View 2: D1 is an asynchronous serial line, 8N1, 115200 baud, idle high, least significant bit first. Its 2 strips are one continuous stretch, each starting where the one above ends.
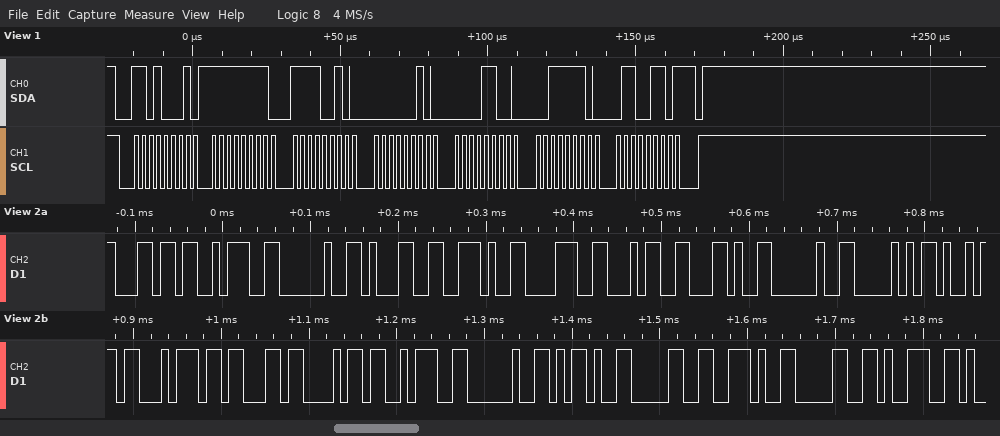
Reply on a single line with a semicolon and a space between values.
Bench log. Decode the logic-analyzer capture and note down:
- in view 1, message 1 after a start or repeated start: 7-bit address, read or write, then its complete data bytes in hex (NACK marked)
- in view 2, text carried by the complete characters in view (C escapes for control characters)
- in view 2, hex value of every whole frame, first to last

0x68 read: FF F2 02 0C 3E 66 NACK; "l: 1.84, Pitch: -0.09"; 0x6C 0x3A 0x20 0x31 0x2E 0x38 0x34 0x2C 0x20 0x50 0x69 0x74 0x63 0x68 0x3A 0x20 0x2D 0x30 0x2E 0x30 0x39
